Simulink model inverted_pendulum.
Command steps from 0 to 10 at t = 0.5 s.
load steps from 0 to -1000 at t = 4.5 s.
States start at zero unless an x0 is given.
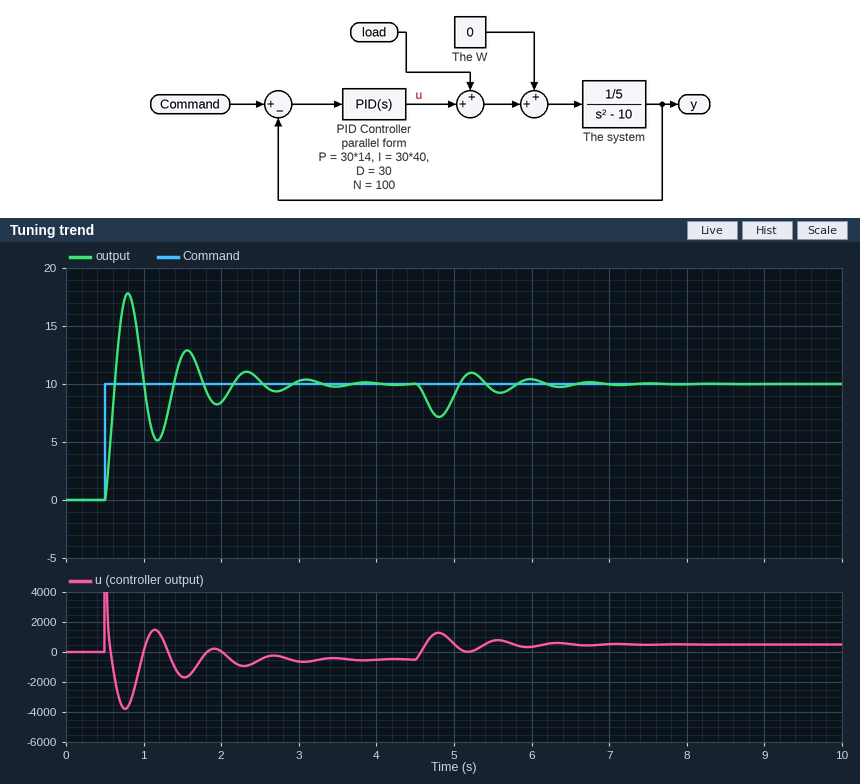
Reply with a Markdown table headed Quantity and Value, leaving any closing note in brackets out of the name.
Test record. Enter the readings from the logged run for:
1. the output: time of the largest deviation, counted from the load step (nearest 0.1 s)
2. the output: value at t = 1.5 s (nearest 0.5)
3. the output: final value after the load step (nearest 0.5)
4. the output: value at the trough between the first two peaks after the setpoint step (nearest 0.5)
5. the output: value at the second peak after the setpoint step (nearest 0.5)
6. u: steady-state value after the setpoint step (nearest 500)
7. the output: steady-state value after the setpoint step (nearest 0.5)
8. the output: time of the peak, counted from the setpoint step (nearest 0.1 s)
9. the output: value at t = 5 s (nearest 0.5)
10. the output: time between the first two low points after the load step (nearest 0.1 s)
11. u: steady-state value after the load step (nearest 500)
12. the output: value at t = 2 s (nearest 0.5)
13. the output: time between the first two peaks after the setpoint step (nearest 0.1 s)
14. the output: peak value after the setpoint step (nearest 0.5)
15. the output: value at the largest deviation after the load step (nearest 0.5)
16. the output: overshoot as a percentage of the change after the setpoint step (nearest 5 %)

| Quantity | Value |
|---|---|
| the output: time of the largest deviation, counted from the load step | 0.3 s |
| the output: value at t = 1.5 s | 12.5 |
| the output: final value after the load step | 10.0 |
| the output: value at the trough between the first two peaks after the setpoint step | 5.0 |
| the output: value at the second peak after the setpoint step | 13.0 |
| u: steady-state value after the setpoint step | -500 |
| the output: steady-state value after the setpoint step | 10.0 |
| the output: time of the peak, counted from the setpoint step | 0.3 s |
| the output: value at t = 5 s | 9.0 |
| the output: time between the first two low points after the load step | 0.8 s |
| u: steady-state value after the load step | 500 |
| the output: value at t = 2 s | 8.5 |
| the output: time between the first two peaks after the setpoint step | 0.8 s |
| the output: peak value after the setpoint step | 18.0 |
| the output: value at the largest deviation after the load step | 7.0 |
| the output: overshoot as a percentage of the change after the setpoint step | 80 % |
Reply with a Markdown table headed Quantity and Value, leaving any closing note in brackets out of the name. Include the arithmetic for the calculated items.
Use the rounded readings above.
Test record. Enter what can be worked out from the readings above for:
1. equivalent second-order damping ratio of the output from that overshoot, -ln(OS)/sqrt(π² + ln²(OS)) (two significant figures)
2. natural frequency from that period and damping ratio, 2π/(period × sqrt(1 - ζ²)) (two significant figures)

| Quantity | Value |
|---|---|
| equivalent second-order damping ratio of the output from that overshoot, -ln(OS)/sqrt(π² + ln²(OS)) | ln(0.8) = -0.223; 0.223 / sqrt(9.870 + 0.050) = 0.071 |
| natural frequency from that period and damping ratio, 2π/(period × sqrt(1 - ζ²)) | 2π / (0.8 × sqrt(1 - 0.071²)) = 7.9 rad/s |
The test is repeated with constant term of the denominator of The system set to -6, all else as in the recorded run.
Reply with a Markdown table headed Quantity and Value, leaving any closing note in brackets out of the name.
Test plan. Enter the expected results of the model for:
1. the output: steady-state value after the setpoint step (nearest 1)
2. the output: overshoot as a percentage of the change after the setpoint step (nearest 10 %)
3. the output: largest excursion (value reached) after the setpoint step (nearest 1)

| Quantity | Value |
|---|---|
| the output: steady-state value after the setpoint step | 10 |
| the output: overshoot as a percentage of the change after the setpoint step | 70 % |
| the output: largest excursion (value reached) after the setpoint step | 17 |
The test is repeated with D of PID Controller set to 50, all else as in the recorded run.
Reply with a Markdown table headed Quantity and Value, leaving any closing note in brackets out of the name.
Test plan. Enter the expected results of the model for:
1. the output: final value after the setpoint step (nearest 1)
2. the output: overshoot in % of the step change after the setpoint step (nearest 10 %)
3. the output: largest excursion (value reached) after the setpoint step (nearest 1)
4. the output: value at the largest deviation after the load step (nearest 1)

| Quantity | Value |
|---|---|
| the output: final value after the setpoint step | 10 |
| the output: overshoot in % of the step change after the setpoint step | 50 % |
| the output: largest excursion (value reached) after the setpoint step | 15 |
| the output: value at the largest deviation after the load step | 8 |
